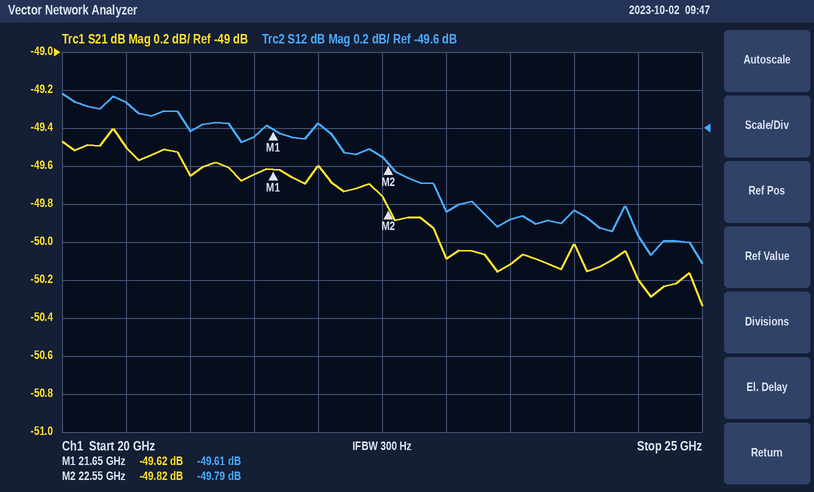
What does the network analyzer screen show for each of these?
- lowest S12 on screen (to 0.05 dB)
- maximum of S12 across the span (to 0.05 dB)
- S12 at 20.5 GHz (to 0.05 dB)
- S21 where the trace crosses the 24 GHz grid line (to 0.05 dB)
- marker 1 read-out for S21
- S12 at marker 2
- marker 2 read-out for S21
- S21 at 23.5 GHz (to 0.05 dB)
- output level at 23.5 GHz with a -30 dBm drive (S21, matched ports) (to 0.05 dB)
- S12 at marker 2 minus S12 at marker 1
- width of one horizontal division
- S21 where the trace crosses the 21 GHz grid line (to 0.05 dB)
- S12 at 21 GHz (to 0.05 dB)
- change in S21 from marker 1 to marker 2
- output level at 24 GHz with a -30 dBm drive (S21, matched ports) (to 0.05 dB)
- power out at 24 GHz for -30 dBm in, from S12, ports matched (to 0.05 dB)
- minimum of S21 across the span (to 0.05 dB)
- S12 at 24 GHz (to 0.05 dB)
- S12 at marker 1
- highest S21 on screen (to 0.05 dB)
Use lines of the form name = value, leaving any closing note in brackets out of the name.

lowest S12 on screen = -50.30 dB
maximum of S12 across the span = -49.40 dB
S12 at 20.5 GHz = -49.45 dB
S21 where the trace crosses the 24 GHz grid line = -50.00 dB
marker 1 read-out for S21 = -49.62 dB
S12 at marker 2 = -49.79 dB
marker 2 read-out for S21 = -49.82 dB
S21 at 23.5 GHz = -50.10 dB
output level at 23.5 GHz with a -30 dBm drive (S21, matched ports) = -80.10 dBm
S12 at marker 2 minus S12 at marker 1 = -0.18 dB
width of one horizontal division = 500 MHz
S21 where the trace crosses the 21 GHz grid line = -49.65 dB
S12 at 21 GHz = -49.60 dB
change in S21 from marker 1 to marker 2 = -0.20 dB
output level at 24 GHz with a -30 dBm drive (S21, matched ports) = -80.00 dBm
power out at 24 GHz for -30 dBm in, from S12, ports matched = -80.05 dBm
minimum of S21 across the span = -50.35 dB
S12 at 24 GHz = -50.05 dB
S12 at marker 1 = -49.61 dB
highest S21 on screen = -49.40 dB
